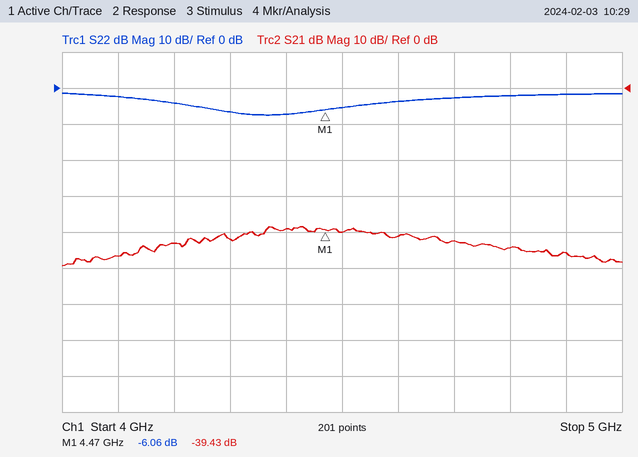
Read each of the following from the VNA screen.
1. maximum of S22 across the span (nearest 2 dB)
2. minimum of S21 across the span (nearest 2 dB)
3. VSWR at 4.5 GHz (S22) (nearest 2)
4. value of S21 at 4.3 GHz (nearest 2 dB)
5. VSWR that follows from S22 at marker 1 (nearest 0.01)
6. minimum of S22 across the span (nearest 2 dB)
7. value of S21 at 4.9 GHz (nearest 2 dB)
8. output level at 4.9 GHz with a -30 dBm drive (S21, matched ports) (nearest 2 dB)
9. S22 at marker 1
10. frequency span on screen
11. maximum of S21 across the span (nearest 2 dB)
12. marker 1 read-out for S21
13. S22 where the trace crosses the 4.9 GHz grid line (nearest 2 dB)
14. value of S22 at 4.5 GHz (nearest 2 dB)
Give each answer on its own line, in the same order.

-2 dB
-50 dB
4
-42 dB
2.98
-8 dB
-46 dB
-76 dBm
-6.06 dB
1 GHz
-38 dB
-39.43 dB
-2 dB
-6 dB
